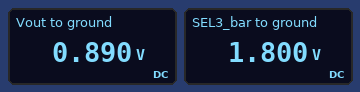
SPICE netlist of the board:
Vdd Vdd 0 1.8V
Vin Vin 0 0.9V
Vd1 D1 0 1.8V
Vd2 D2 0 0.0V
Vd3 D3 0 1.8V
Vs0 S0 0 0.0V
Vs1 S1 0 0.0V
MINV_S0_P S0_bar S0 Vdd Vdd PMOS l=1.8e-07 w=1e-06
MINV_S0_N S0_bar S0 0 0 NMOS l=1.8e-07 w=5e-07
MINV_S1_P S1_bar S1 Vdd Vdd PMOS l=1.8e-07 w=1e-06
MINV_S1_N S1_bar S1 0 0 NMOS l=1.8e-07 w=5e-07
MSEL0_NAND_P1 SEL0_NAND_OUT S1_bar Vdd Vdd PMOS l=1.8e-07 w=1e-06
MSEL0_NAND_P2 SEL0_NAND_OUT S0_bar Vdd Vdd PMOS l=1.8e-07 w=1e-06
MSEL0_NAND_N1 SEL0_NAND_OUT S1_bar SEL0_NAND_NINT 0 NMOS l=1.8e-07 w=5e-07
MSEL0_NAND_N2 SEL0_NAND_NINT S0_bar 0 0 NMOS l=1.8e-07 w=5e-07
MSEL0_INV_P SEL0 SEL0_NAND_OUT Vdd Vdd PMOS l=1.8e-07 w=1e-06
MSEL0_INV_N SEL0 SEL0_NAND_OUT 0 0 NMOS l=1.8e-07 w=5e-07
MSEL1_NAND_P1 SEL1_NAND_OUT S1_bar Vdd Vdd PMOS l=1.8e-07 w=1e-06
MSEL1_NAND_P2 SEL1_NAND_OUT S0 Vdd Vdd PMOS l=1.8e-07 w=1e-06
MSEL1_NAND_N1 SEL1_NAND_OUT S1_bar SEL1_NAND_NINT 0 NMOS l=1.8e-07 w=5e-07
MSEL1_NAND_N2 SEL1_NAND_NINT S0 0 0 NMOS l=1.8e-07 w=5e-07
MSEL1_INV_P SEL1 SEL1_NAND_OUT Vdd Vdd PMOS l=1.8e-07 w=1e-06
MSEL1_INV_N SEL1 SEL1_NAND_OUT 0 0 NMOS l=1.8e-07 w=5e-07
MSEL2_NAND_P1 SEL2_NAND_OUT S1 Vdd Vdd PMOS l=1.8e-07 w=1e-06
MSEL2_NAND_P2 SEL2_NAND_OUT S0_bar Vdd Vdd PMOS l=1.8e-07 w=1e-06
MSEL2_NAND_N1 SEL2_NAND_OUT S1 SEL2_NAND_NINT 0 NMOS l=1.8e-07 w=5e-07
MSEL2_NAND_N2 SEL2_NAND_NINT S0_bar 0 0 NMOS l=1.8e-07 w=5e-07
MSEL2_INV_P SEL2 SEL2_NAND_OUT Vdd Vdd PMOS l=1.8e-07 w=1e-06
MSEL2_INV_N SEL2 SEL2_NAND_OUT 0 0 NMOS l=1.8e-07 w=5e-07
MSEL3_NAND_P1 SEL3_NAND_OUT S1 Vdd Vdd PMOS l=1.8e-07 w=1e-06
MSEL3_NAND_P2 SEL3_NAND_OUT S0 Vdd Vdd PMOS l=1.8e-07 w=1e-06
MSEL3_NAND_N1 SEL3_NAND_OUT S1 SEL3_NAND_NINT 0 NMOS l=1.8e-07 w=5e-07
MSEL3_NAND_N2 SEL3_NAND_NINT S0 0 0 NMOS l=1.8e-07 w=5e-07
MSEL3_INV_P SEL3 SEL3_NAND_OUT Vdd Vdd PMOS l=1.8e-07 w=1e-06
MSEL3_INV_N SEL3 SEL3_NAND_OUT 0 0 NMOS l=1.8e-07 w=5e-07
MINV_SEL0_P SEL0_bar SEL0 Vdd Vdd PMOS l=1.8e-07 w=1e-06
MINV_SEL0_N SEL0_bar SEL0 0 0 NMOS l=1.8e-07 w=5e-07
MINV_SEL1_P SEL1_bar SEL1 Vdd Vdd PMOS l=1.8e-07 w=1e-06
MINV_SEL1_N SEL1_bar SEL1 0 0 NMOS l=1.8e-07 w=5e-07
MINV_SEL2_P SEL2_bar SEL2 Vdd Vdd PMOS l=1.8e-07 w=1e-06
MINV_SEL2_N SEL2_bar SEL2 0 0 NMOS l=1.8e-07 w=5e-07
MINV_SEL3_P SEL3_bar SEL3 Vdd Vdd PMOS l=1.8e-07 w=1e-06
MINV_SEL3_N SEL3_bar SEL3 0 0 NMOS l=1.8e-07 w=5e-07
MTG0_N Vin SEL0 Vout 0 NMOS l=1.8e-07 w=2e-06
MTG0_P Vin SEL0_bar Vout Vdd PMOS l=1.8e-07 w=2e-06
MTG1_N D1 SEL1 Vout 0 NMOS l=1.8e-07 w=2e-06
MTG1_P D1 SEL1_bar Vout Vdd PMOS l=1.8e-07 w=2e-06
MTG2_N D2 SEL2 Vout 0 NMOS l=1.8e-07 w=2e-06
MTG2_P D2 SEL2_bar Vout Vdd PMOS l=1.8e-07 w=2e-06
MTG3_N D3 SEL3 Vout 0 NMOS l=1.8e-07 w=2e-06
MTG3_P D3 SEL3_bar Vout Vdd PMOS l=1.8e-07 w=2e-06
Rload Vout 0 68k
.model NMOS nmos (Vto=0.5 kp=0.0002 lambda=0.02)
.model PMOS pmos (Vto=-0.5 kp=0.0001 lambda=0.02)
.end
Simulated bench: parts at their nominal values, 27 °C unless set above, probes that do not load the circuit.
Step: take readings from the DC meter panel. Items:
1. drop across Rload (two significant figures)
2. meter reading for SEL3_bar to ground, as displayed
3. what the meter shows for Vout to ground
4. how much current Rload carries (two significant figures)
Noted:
890 mV
1.800 V
0.890 V
13 µA
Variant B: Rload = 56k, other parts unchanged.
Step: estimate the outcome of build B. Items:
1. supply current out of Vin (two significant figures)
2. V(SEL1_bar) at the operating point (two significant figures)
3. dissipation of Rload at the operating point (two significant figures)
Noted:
16 µA
1.8 V
14 µW
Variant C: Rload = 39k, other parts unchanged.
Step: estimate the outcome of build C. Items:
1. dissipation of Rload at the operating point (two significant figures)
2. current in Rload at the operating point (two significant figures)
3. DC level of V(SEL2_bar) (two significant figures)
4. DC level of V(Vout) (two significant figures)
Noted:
20 µW
23 µA
1.8 V
880 mV
